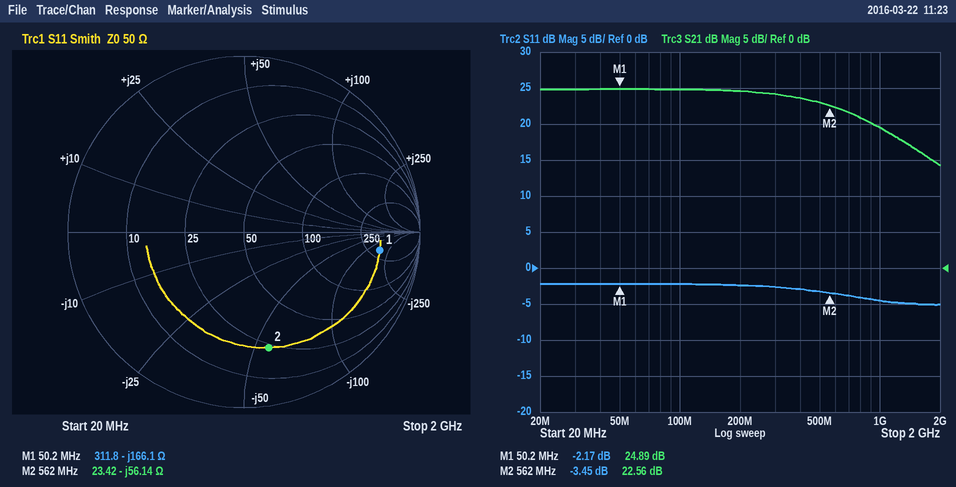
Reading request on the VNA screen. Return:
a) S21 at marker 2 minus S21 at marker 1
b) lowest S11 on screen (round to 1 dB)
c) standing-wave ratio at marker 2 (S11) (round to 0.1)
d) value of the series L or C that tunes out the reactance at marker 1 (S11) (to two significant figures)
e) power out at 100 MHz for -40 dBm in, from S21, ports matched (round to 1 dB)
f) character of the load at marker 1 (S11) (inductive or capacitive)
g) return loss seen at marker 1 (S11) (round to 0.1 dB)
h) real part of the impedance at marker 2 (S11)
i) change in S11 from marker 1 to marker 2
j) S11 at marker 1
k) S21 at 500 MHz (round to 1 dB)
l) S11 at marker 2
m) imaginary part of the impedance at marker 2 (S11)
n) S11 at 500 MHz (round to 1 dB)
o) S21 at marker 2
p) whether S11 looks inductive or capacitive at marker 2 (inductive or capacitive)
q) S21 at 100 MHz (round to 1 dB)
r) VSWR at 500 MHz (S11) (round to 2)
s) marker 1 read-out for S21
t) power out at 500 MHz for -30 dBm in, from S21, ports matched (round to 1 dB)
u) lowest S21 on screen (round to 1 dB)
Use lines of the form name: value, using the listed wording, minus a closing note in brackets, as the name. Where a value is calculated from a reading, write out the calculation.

S21 at marker 2 minus S21 at marker 1: 22.56 − (24.89) = -2.33 dB
lowest S11 on screen: -5 dB
standing-wave ratio at marker 2 (S11): 5.1
value of the series L or C that tunes out the reactance at marker 1 (S11): L = 166.1 Ω/(2π × 50.2 MHz) ≈ 527 nH, so 530 nH to two significant figures
power out at 100 MHz for -40 dBm in, from S21, ports matched: -40 dBm + (25 dB) = -15 dBm
character of the load at marker 1 (S11): capacitive
return loss seen at marker 1 (S11): 2.2 dB
real part of the impedance at marker 2: 23.42 Ω
change in S11 from marker 1 to marker 2: -3.45 − (-2.17) = -1.28 dB
S11 at marker 1: -2.17 dB
S21 at 500 MHz: 23 dB
S11 at marker 2: -3.45 dB
imaginary part of the impedance at marker 2: -56.14 Ω
S11 at 500 MHz: -3 dB
S21 at marker 2: 22.56 dB
whether S11 looks inductive or capacitive at marker 2: capacitive
S21 at 100 MHz: 25 dB
VSWR at 500 MHz (S11): |Γ| = 10^(-3/20) = 0.7079; VSWR = (1 + 0.7079)/(1 − 0.7079) ≈ 6
marker 1 read-out for S21: 24.89 dB
power out at 500 MHz for -30 dBm in, from S21, ports matched: -30 dBm + (23 dB) = -7 dBm
lowest S21 on screen: 14 dB
